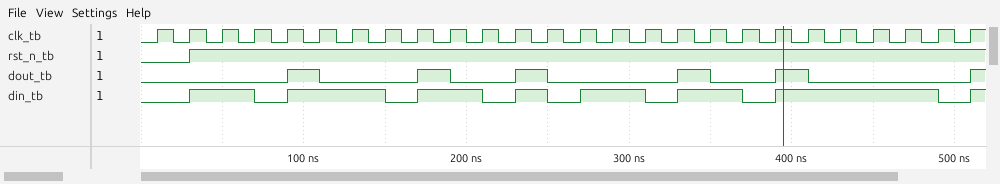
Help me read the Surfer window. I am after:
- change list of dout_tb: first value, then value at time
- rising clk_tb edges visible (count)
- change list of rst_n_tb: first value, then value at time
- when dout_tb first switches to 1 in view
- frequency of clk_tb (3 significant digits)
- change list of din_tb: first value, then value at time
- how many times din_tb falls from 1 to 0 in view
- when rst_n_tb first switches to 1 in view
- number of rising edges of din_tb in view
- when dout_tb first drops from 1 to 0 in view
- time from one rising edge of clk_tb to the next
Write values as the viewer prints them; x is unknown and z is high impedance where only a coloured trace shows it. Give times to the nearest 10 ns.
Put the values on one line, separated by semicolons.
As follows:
0, 1 at 90 ns, 0 at 110 ns, 1 at 170 ns, 0 at 190 ns, 1 at 230 ns, 0 at 250 ns, 1 at 330 ns, 0 at 350 ns, 1 at 390 ns, 0 at 410 ns, 1 at 510 ns; 26; 0, 1 at 30 ns; 90 ns; 50.0 MHz; 0, 1 at 30 ns, 0 at 70 ns, 1 at 90 ns, 0 at 150 ns, 1 at 170 ns, 0 at 210 ns, 1 at 230 ns, 0 at 250 ns, 1 at 270 ns, 0 at 310 ns, 1 at 330 ns, 0 at 370 ns, 1 at 390 ns, 0 at 490 ns, 1 at 510 ns; 7; 30 ns; 8; 110 ns; 20 ns
